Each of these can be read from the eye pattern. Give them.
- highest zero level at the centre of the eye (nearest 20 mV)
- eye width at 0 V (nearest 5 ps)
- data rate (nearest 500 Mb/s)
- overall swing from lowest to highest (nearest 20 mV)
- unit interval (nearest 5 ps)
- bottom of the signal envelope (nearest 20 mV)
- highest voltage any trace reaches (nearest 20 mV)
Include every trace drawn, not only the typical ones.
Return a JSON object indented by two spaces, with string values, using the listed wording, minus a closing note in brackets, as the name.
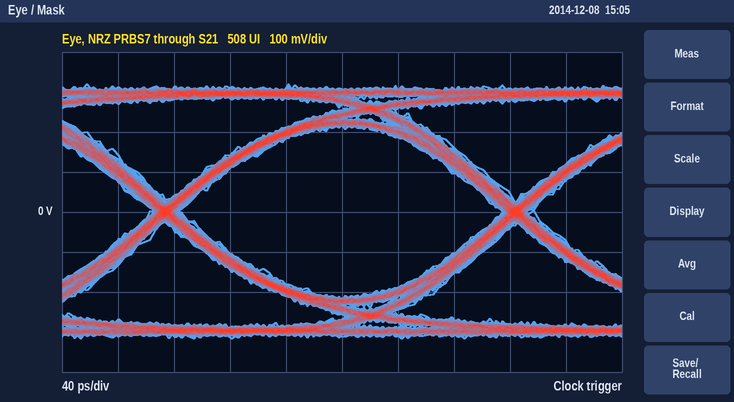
{
  "highest zero level at the centre of the eye": "-220 mV",
  "eye width at 0 V": "230 ps",
  "data rate": "4.0 Gb/s",
  "overall swing from lowest to highest": "640 mV",
  "unit interval": "250 ps",
  "bottom of the signal envelope": "-320 mV",
  "highest voltage any trace reaches": "320 mV"
}
